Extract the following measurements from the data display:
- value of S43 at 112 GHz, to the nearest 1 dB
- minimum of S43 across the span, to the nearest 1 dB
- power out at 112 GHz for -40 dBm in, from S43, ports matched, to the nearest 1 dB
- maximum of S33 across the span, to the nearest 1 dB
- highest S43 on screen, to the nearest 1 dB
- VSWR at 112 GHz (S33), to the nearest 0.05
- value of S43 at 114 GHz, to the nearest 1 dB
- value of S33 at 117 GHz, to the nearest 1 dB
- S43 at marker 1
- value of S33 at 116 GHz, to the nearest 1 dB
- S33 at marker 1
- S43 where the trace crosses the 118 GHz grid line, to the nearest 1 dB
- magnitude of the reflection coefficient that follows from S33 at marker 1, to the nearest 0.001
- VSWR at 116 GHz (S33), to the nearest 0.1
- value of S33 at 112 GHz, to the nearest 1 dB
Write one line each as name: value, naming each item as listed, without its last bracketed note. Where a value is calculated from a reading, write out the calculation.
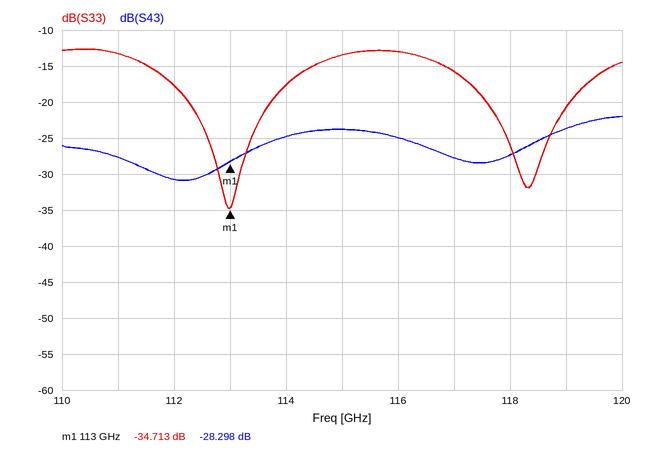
value of S43 at 112 GHz, to the nearest 1 dB: -31 dB
minimum of S43 across the span, to the nearest 1 dB: -31 dB
power out at 112 GHz for -40 dBm in, from S43, ports matched, to the nearest 1 dB: -40 dBm + (-31 dB) = -71 dBm
maximum of S33 across the span, to the nearest 1 dB: -13 dB
highest S43 on screen, to the nearest 1 dB: -22 dB
VSWR at 112 GHz (S33), to the nearest 0.05: |Γ| = 10^(-18/20) = 0.1259; VSWR = (1 + 0.1259)/(1 − 0.1259) ≈ 1.29, so 1.30 to the nearest 0.05
value of S43 at 114 GHz, to the nearest 1 dB: -25 dB
value of S33 at 117 GHz, to the nearest 1 dB: -16 dB
S43 at marker 1: -28.298 dB
value of S33 at 116 GHz, to the nearest 1 dB: -13 dB
S33 at marker 1: -34.713 dB
S43 where the trace crosses the 118 GHz grid line, to the nearest 1 dB: -27 dB
magnitude of the reflection coefficient that follows from S33 at marker 1, to the nearest 0.001: 10^(-34.713/20) ≈ 0.018
VSWR at 116 GHz (S33), to the nearest 0.1: |Γ| = 10^(-13/20) = 0.2239; VSWR = (1 + 0.2239)/(1 − 0.2239) ≈ 1.6
value of S33 at 112 GHz, to the nearest 1 dB: -18 dB
